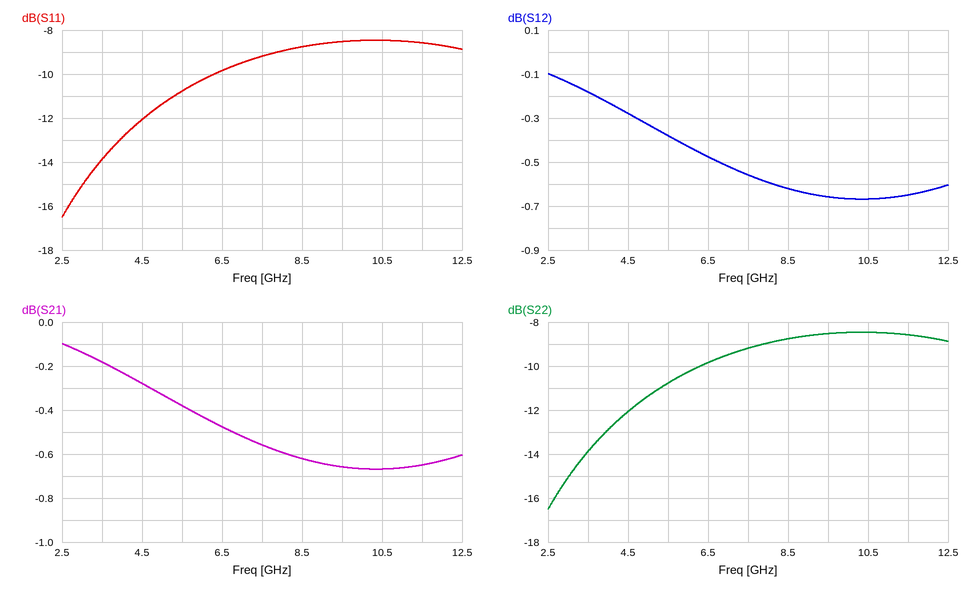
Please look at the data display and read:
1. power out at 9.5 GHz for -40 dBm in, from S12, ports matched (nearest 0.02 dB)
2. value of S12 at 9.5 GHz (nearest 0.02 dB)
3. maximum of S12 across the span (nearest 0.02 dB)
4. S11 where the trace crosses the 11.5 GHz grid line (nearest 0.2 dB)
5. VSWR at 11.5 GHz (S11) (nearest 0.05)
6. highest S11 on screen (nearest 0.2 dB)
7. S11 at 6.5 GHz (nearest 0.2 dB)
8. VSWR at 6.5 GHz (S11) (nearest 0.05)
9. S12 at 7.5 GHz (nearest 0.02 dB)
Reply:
-40.66 dBm
-0.66 dB
-0.10 dB
-8.6 dB
2.20
-8.4 dB
-9.8 dB
1.95
-0.56 dB
